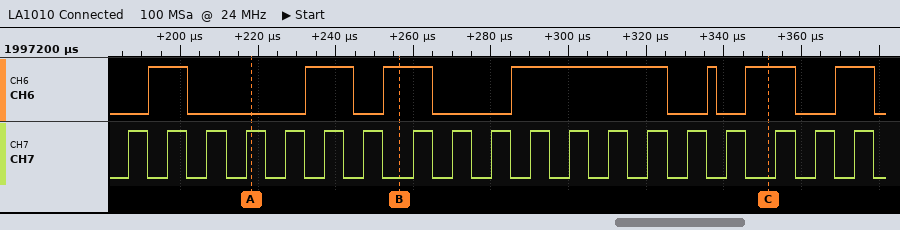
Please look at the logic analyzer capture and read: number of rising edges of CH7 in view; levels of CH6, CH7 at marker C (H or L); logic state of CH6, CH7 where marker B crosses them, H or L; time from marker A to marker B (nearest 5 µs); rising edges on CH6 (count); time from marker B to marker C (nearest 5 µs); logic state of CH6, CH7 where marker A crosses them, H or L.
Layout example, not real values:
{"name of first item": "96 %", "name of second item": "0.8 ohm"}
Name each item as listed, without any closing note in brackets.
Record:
{"number of rising edges of CH7 in view": "19", "levels of CH6, CH7 at marker C": "CH6=H, CH7=L", "logic state of CH6, CH7 where marker B crosses them, H or L": "CH6=H, CH7=L", "time from marker A to marker B": "40 µs", "rising edges on CH6": "7", "time from marker B to marker C": "95 µs", "logic state of CH6, CH7 where marker A crosses them, H or L": "CH6=L, CH7=H"}
